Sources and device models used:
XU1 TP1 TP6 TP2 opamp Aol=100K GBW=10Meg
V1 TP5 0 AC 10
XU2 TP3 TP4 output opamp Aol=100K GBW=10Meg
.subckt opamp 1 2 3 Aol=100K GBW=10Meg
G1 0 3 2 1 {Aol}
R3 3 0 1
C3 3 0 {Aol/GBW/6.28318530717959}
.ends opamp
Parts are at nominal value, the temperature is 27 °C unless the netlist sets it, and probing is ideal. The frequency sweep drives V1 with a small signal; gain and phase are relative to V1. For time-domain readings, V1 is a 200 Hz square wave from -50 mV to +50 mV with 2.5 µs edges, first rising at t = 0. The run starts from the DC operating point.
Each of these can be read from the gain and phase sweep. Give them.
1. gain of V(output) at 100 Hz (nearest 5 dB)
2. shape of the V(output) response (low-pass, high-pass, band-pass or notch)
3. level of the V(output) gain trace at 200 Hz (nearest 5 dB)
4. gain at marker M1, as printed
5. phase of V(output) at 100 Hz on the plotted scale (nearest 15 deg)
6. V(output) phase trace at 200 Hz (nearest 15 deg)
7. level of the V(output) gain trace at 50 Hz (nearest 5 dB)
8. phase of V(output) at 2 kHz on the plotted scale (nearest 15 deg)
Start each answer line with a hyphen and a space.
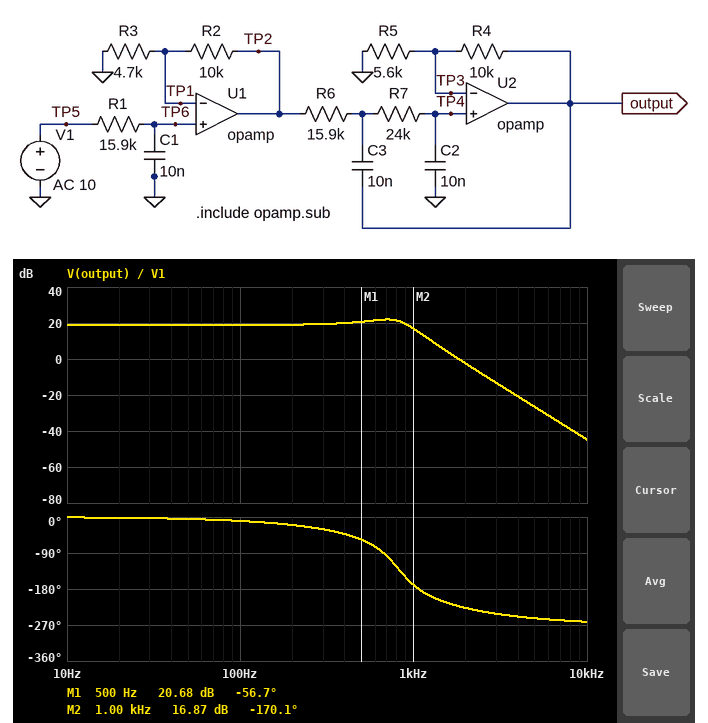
- 20 dB
- low-pass
- 20 dB
- 20.68 dB
- -15 deg
- -15 deg
- 20 dB
- -225 deg
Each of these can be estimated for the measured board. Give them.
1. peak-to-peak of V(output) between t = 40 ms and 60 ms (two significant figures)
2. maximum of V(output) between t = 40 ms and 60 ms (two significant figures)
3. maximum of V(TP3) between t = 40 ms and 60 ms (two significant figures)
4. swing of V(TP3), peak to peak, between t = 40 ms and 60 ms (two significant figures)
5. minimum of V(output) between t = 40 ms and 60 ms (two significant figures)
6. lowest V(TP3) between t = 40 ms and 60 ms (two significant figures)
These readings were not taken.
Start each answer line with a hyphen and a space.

- 1.3 V
- 670 mV
- 240 mV
- 480 mV
- -670 mV
- -240 mV
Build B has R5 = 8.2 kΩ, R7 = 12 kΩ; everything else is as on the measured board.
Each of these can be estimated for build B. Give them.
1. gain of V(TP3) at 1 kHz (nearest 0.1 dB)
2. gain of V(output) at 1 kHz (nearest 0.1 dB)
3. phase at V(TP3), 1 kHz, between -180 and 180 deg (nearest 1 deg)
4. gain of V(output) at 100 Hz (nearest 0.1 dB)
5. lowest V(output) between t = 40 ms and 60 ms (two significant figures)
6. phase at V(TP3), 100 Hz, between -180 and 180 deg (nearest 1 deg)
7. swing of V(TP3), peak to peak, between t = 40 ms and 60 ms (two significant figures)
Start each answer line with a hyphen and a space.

- 11.5 dB
- 18.4 dB
- -110 deg
- 16.8 dB
- -480 mV
- -9 deg
- 430 mV
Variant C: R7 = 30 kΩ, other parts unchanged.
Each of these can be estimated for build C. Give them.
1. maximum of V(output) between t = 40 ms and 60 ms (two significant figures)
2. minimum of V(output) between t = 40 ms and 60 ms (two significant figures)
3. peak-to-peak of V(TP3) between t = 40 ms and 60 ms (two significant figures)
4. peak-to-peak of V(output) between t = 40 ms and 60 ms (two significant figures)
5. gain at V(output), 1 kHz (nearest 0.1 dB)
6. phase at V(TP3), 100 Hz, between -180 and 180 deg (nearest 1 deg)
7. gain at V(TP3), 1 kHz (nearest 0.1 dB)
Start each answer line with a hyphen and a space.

- 600 mV
- -600 mV
- 430 mV
- 1.2 V
- 12.8 dB
- -12 deg
- 3.9 dB
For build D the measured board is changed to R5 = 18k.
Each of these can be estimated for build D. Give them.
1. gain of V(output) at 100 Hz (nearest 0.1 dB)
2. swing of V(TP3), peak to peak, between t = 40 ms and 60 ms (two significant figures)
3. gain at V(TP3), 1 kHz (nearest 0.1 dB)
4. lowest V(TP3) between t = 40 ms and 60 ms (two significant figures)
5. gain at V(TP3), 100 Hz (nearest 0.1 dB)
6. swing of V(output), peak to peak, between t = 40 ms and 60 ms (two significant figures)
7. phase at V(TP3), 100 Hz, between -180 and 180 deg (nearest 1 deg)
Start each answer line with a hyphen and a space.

- 13.7 dB
- 320 mV
- 0.8 dB
- -160 mV
- 9.8 dB
- 490 mV
- -17 deg
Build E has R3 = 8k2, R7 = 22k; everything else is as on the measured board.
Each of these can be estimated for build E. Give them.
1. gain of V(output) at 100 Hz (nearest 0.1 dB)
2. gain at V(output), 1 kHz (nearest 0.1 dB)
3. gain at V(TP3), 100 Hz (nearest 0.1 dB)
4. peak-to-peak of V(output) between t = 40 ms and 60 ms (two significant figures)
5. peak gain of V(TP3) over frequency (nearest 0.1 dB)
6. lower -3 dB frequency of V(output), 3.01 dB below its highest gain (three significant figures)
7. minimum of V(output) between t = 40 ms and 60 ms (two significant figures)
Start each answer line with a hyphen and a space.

- 15.9 dB
- 15.8 dB
- 7.0 dB
- 990 mV
- 11.0 dB
- 393 Hz
- -490 mV
